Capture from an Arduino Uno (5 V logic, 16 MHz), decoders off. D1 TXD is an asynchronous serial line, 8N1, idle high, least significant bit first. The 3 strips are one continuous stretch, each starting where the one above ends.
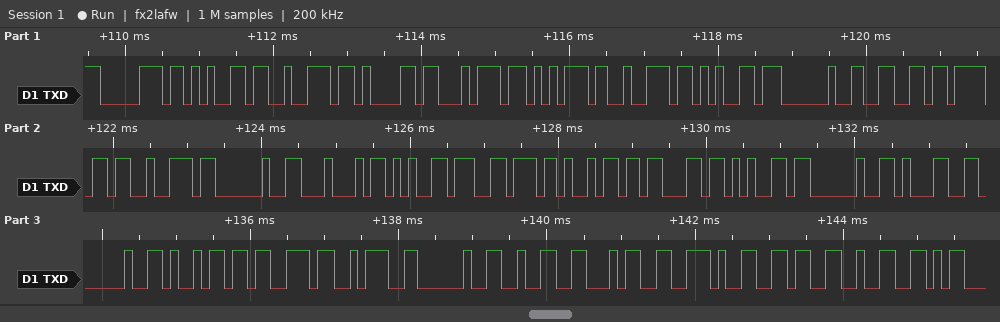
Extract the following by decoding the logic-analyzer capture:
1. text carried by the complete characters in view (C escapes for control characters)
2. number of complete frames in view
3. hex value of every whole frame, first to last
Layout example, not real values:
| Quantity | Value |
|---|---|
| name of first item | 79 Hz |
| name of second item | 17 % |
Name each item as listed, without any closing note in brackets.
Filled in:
| Quantity | Value |
|---|---|
| text carried by the complete characters in view | "perature for Device 1 is: 24.62" |
| number of complete frames in view | 31 |
| hex value of every whole frame, first to last | 0x70 0x65 0x72 0x61 0x74 0x75 0x72 0x65 0x20 0x66 0x6F 0x72 0x20 0x44 0x65 0x76 0x69 0x63 0x65 0x20 0x31 0x20 0x69 0x73 0x3A 0x20 0x32 0x34 0x2E 0x36 0x32 |
